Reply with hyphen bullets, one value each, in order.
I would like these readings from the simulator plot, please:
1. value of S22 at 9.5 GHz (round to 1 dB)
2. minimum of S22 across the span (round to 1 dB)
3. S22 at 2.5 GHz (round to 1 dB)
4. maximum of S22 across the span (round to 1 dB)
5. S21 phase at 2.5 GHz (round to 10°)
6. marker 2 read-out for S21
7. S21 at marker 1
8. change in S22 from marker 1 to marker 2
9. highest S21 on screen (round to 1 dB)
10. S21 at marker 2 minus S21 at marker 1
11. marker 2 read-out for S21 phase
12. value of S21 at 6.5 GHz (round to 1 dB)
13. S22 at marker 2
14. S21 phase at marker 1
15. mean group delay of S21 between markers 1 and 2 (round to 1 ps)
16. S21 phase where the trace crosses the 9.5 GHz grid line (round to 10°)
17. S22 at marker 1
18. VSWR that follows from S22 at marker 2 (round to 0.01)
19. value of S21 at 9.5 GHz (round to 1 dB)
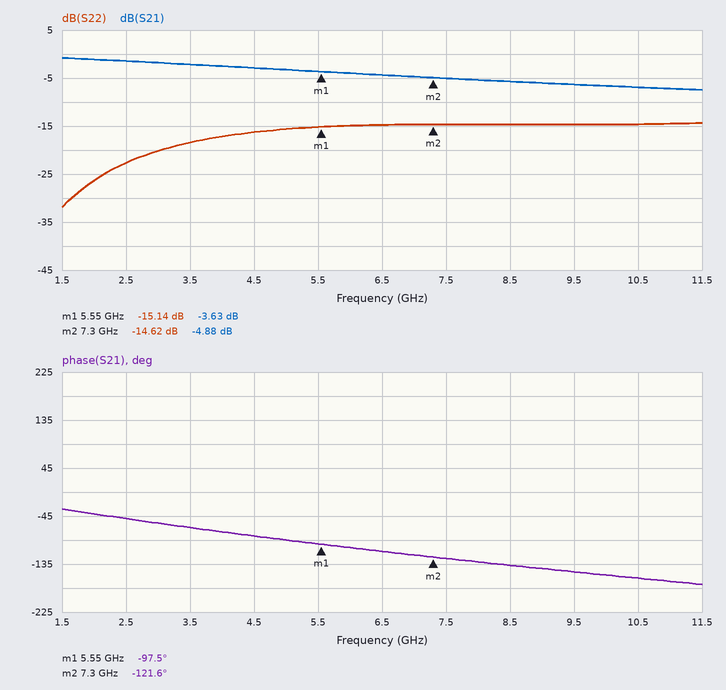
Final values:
- -15 dB
- -32 dB
- -23 dB
- -14 dB
- -50°
- -4.88 dB
- -3.63 dB
- 0.52 dB
- -1 dB
- -1.25 dB
- -121.6°
- -4 dB
- -14.62 dB
- -97.5°
- 38 ps
- -150°
- -15.14 dB
- 1.46
- -6 dB
